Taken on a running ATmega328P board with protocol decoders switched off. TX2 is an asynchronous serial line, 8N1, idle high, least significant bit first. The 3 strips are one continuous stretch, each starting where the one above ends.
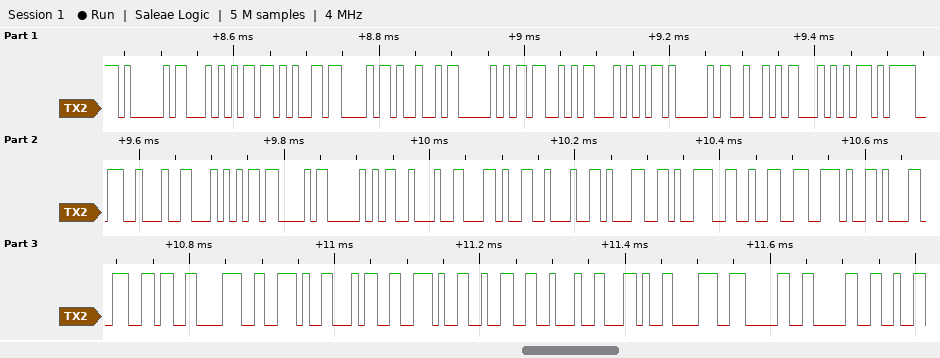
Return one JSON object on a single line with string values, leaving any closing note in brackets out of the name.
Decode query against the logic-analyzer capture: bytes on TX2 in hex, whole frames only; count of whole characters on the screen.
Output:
{"bytes on TX2 in hex, whole frames only": "41 54 2B 43 49 50 53 54 41 52 54 3D 22 54 43 50 22 2C 22 31 39 32 2E 31 36 38 2E 34 2E 32 22 2C 38 30 30", "count of whole characters on the screen": "35"}
